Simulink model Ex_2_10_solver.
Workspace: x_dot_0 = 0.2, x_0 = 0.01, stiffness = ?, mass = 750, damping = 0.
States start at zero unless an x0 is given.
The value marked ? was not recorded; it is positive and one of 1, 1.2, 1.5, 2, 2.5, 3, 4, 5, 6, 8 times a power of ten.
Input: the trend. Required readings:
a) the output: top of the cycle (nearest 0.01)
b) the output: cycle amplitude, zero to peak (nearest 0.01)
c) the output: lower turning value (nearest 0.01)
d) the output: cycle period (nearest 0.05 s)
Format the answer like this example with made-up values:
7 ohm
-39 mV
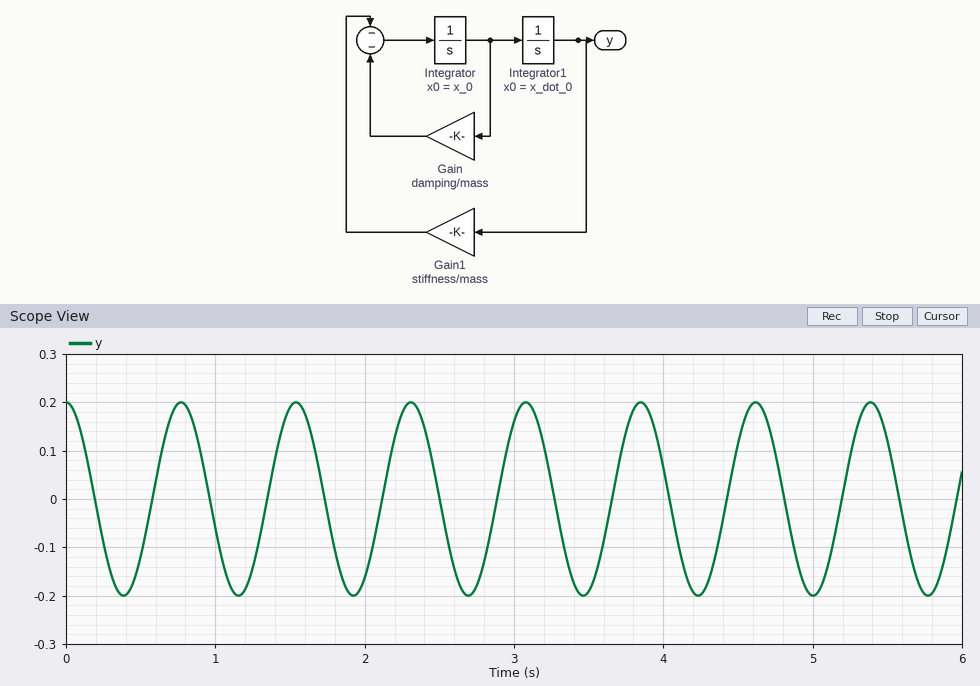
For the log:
0.20
0.20
-0.20
0.75 s
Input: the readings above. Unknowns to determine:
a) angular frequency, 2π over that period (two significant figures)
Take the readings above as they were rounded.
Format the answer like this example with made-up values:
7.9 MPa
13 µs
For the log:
8.4 rad/s
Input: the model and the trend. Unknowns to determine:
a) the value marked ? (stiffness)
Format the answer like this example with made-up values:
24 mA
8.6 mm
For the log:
50000
